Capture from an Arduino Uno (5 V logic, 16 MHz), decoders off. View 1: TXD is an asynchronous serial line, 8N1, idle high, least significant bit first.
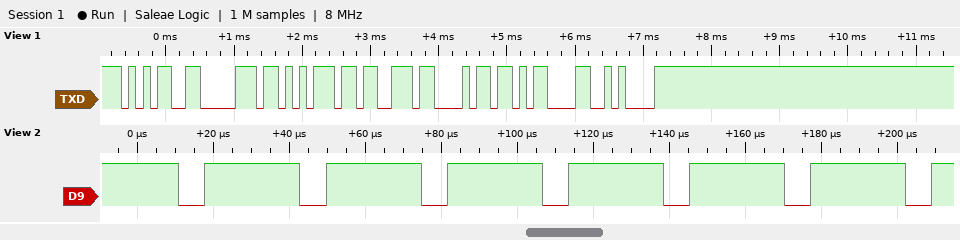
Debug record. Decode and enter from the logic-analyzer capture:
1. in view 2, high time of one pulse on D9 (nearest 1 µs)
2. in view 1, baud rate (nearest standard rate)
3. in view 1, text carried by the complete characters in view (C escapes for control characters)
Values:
25 µs
9600 baud
"5push\r\n"
